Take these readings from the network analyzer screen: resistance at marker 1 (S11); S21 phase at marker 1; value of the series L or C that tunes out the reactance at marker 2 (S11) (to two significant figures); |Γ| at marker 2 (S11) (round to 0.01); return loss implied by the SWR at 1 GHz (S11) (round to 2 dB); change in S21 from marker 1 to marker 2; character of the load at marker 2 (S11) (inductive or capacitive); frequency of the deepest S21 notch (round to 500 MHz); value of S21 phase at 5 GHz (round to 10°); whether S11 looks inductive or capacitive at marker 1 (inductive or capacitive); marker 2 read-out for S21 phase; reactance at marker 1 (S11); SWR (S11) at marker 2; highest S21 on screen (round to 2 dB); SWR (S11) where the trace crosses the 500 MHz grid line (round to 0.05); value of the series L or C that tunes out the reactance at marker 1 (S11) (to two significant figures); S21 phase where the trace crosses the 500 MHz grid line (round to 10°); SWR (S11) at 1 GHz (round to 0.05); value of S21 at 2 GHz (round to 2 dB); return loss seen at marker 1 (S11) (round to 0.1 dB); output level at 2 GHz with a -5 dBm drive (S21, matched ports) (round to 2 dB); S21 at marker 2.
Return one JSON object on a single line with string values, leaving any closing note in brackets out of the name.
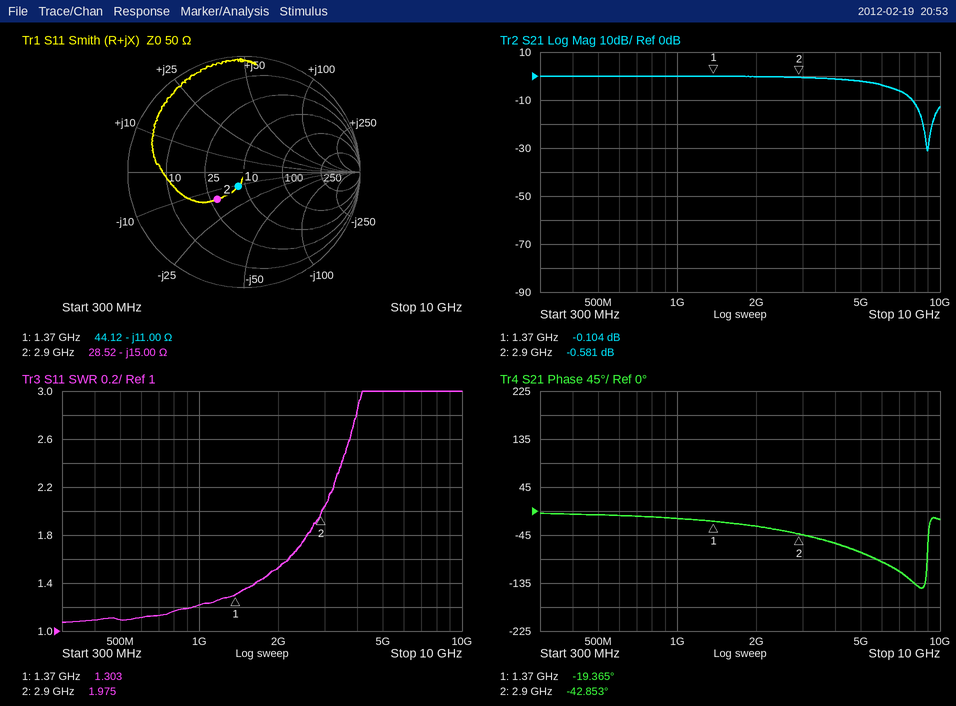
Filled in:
{"resistance at marker 1": "44.12 Ω", "S21 phase at marker 1": "-19.365°", "value of the series L or C that tunes out the reactance at marker 2 (S11)": "820 pH", "|Γ| at marker 2 (S11)": "0.33", "return loss implied by the SWR at 1 GHz (S11)": "20 dB", "change in S21 from marker 1 to marker 2": "-0.477 dB", "character of the load at marker 2 (S11)": "capacitive", "frequency of the deepest S21 notch": "9.0 GHz", "value of S21 phase at 5 GHz": "-80°", "whether S11 looks inductive or capacitive at marker 1": "capacitive", "marker 2 read-out for S21 phase": "-42.853°", "reactance at marker 1": "-11.00 Ω", "SWR (S11) at marker 2": "1.975", "highest S21 on screen": "0 dB", "SWR (S11) where the trace crosses the 500 MHz grid line": "1.10", "value of the series L or C that tunes out the reactance at marker 1 (S11)": "1.3 nH", "S21 phase where the trace crosses the 500 MHz grid line": "-10°", "SWR (S11) at 1 GHz": "1.20", "value of S21 at 2 GHz": "0 dB", "return loss seen at marker 1 (S11)": "17.6 dB", "output level at 2 GHz with a -5 dBm drive (S21, matched ports)": "-6 dBm", "S21 at marker 2": "-0.581 dB"}
